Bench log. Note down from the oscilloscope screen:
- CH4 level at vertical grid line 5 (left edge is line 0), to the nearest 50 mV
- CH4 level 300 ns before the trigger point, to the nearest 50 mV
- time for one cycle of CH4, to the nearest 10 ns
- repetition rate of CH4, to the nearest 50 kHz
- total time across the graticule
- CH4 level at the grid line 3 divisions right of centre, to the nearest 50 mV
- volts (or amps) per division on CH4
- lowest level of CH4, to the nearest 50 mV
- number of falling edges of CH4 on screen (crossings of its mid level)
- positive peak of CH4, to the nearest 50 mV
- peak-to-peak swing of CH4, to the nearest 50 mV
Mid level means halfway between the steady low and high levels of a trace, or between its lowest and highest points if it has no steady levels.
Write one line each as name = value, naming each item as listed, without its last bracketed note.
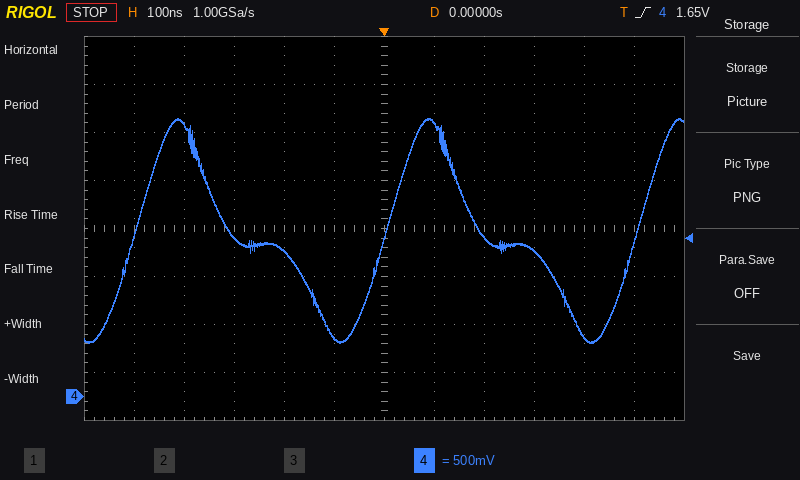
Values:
CH4 level at vertical grid line 5 (left edge is line 0), to the nearest 50 mV = 600 mV
CH4 level 300 ns before the trigger point, to the nearest 50 mV = 1.65 V
time for one cycle of CH4, to the nearest 10 ns = 500 ns
repetition rate of CH4, to the nearest 50 kHz = 2.00 MHz
total time across the graticule = 1.2 µs
CH4 level at the grid line 3 divisions right of centre, to the nearest 50 mV = 1.50 V
volts (or amps) per division on CH4 = 500 mV
lowest level of CH4, to the nearest 50 mV = 550 mV
number of falling edges of CH4 on screen = 2
positive peak of CH4, to the nearest 50 mV = 2.90 V
peak-to-peak swing of CH4, to the nearest 50 mV = 2.35 V
